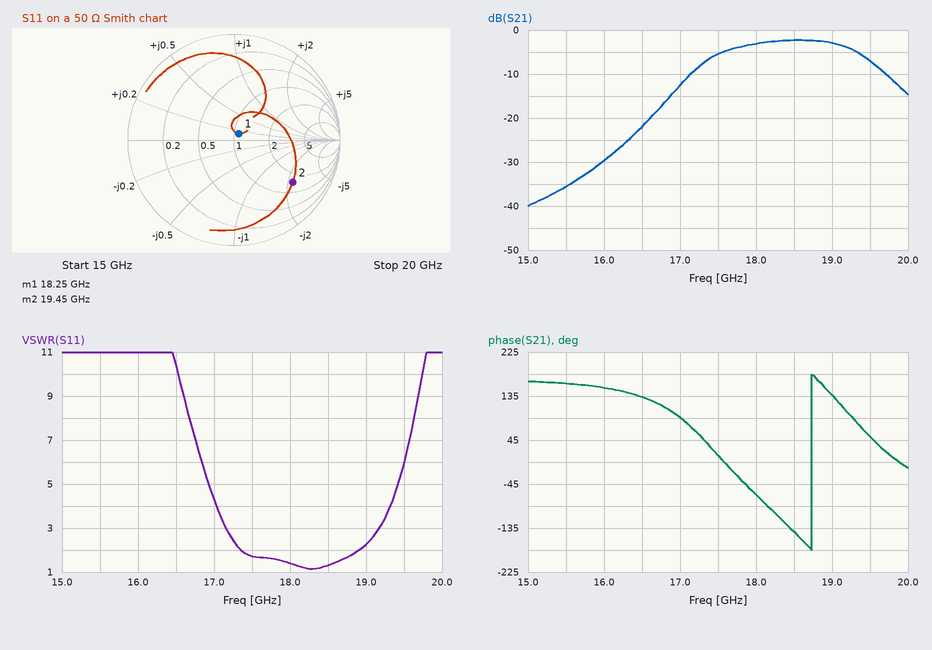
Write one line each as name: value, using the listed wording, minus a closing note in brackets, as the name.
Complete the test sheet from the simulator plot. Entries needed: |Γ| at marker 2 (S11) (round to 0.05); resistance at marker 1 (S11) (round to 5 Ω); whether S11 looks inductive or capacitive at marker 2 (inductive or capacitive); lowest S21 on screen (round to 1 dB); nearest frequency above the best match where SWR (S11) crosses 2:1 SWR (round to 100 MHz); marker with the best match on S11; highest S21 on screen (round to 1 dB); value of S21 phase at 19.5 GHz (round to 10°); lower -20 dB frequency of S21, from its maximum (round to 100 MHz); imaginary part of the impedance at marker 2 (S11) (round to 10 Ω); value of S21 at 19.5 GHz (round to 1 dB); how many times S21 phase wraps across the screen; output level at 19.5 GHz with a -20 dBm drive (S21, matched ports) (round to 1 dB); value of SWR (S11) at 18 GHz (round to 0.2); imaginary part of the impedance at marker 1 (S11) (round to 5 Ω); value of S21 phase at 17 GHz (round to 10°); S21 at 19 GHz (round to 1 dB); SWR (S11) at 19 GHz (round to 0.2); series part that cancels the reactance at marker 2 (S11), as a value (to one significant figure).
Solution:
|Γ| at marker 2 (S11): 0.70
resistance at marker 1 (S11): 55 Ω
whether S11 looks inductive or capacitive at marker 2: capacitive
lowest S21 on screen: -40 dB
nearest frequency above the best match where SWR (S11) crosses 2:1 SWR: 18.9 GHz
marker with the best match on S11: marker 1
highest S21 on screen: -2 dB
value of S21 phase at 19.5 GHz: 50°
lower -20 dB frequency of S21, from its maximum: 16.5 GHz
imaginary part of the impedance at marker 2 (S11): -110 Ω
value of S21 at 19.5 GHz: -7 dB
how many times S21 phase wraps across the screen: 1
output level at 19.5 GHz with a -20 dBm drive (S21, matched ports): -27 dBm
value of SWR (S11) at 18 GHz: 1.4
imaginary part of the impedance at marker 1 (S11): +5 Ω
value of S21 phase at 17 GHz: 90°
S21 at 19 GHz: -3 dB
SWR (S11) at 19 GHz: 2.2
series part that cancels the reactance at marker 2 (S11), as a value: 900 pH
